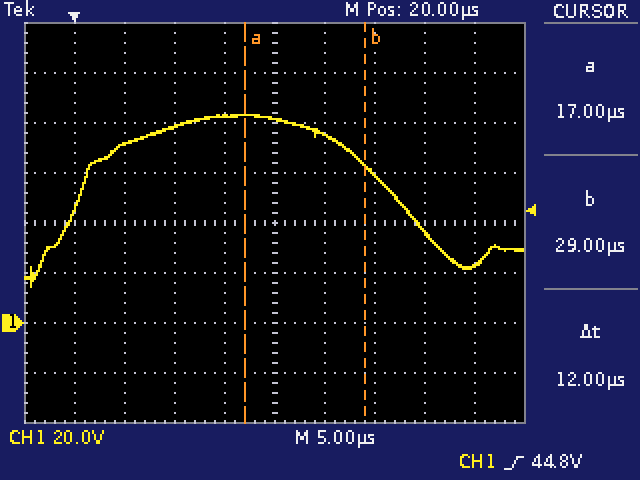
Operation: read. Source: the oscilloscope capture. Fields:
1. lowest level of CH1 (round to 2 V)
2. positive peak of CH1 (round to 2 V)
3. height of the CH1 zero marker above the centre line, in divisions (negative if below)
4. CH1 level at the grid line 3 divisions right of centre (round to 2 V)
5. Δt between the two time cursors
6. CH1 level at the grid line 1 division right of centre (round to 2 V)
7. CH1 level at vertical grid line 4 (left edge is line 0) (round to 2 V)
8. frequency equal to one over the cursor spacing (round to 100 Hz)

14 V
84 V
-2.0 div
36 V
12 µs
76 V
82 V
83.3 kHz
